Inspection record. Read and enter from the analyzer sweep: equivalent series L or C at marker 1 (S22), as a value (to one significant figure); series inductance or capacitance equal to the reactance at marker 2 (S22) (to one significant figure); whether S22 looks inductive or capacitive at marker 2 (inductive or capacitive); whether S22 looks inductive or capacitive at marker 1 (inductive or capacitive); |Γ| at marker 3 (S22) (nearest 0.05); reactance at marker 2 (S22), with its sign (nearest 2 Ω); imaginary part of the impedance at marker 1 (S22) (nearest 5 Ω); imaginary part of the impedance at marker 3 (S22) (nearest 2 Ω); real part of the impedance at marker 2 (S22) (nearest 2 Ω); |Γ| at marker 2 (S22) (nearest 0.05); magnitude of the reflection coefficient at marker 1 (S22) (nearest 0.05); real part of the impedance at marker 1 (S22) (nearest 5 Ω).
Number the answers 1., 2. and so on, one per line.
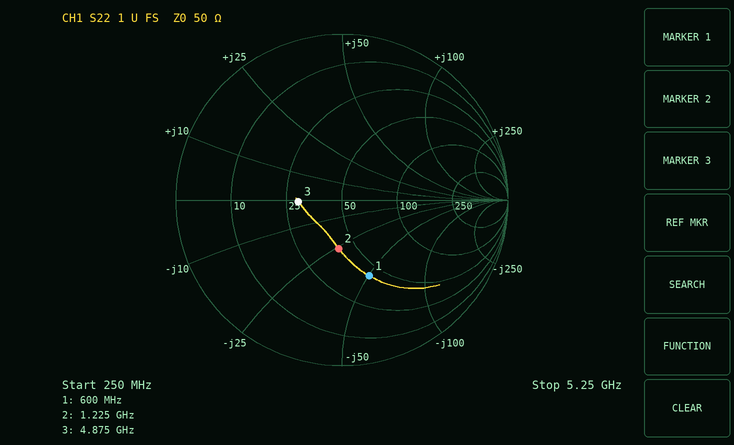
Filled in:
1. 5 pF
2. 5 pF
3. capacitive
4. capacitive
5. 0.25
6. -26 Ω
7. -50 Ω
8. 0 Ω
9. 40 Ω
10. 0.30
11. 0.50
12. 40 Ω
